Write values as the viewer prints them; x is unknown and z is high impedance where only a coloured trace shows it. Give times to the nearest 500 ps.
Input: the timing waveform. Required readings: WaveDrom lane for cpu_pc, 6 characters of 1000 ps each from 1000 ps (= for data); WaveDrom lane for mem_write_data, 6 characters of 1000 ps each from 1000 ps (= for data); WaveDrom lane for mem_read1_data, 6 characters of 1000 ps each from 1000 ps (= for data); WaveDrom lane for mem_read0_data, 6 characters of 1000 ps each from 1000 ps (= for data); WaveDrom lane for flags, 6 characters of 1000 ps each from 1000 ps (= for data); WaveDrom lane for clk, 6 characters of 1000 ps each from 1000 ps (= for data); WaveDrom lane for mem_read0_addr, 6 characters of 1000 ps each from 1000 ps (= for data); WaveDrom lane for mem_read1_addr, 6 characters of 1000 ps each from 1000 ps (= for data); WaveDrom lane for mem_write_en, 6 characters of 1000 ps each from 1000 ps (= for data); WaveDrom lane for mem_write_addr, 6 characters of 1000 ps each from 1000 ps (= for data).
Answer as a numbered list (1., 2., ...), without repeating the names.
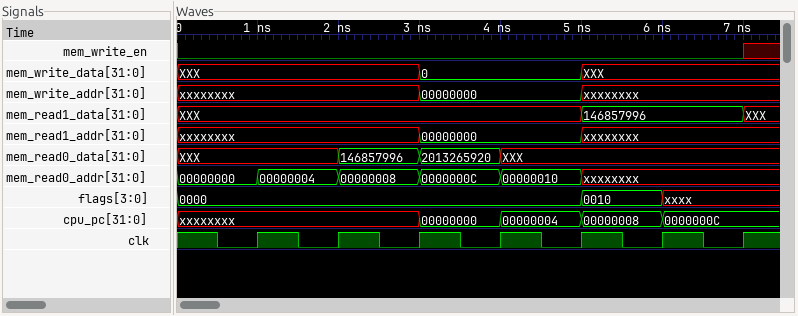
1. {name: 'cpu_pc', wave: 'x.====', data: '00000000 00000004 00000008 0000000C'}
2. {name: 'mem_write_data', wave: 'x.=.x.', data: '0'}
3. {name: 'mem_read1_data', wave: 'x...=.', data: '146857996'}
4. {name: 'mem_read0_data', wave: 'x==x..', data: '146857996 2013265920'}
5. {name: 'flags', wave: '=...=x', data: '0000 0010'}
6. {name: 'clk', wave: 'p.....'}
7. {name: 'mem_read0_addr', wave: '====x.', data: '00000004 00000008 0000000C 00000010'}
8. {name: 'mem_read1_addr', wave: 'x.=.x.', data: '00000000'}
9. {name: 'mem_write_en', wave: '0.....'}
10. {name: 'mem_write_addr', wave: 'x.=.x.', data: '00000000'}
